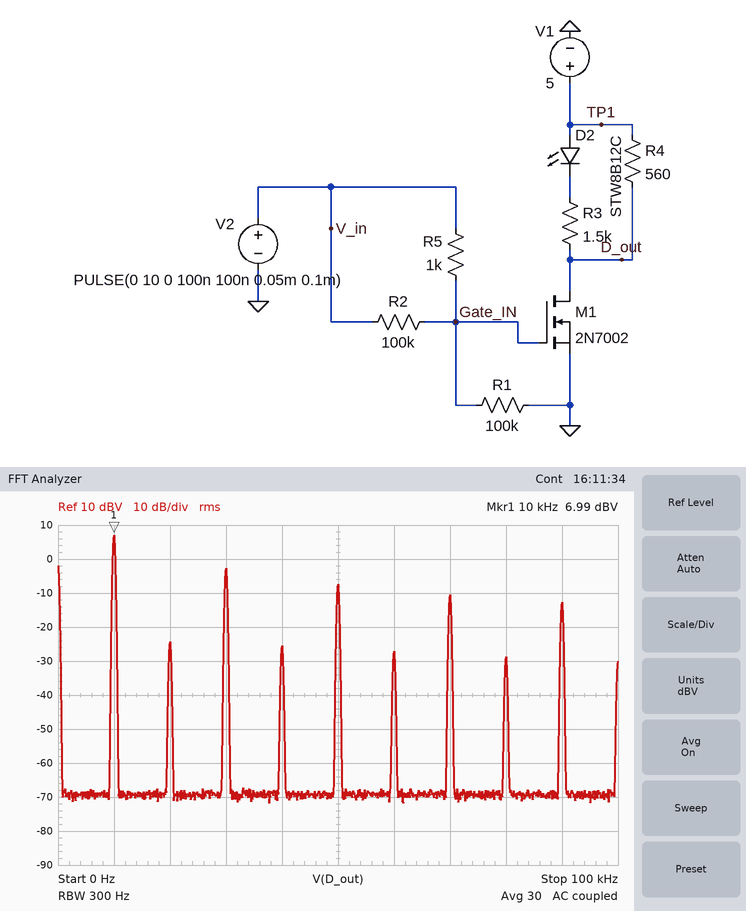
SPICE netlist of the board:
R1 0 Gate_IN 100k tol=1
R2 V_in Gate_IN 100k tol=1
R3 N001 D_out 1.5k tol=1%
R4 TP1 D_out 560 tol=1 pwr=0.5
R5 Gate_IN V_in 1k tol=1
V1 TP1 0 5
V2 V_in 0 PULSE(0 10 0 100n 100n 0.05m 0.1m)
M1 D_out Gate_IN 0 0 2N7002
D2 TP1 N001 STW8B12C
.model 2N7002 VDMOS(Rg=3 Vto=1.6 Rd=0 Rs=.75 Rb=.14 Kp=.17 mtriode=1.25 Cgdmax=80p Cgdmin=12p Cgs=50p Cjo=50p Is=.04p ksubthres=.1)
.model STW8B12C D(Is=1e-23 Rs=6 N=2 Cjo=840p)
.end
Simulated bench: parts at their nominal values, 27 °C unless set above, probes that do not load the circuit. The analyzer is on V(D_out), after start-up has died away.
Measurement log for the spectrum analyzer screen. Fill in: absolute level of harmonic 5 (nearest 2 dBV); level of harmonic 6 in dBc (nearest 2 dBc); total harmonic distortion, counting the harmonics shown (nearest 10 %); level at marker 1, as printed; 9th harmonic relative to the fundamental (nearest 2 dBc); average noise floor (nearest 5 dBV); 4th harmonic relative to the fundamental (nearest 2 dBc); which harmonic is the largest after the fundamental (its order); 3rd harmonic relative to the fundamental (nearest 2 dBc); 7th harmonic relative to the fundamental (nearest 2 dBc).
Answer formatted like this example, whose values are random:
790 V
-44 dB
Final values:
-8 dBV
-34 dBc
40 %
6.99 dBV
-20 dBc
-70 dBV
-32 dBc
3
-10 dBc
-18 dBc
